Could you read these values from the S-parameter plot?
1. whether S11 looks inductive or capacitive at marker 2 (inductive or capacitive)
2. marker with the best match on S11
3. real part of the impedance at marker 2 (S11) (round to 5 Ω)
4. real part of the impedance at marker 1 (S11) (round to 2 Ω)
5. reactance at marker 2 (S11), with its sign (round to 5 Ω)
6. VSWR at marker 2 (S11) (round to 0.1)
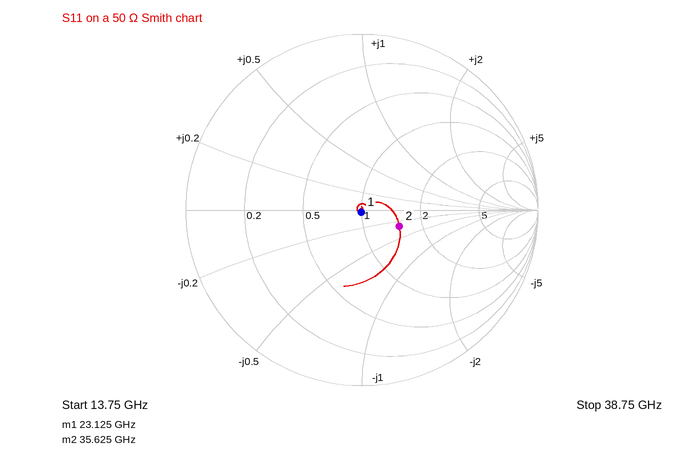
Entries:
capacitive
marker 1
75 Ω
50 Ω
-15 Ω
1.6
